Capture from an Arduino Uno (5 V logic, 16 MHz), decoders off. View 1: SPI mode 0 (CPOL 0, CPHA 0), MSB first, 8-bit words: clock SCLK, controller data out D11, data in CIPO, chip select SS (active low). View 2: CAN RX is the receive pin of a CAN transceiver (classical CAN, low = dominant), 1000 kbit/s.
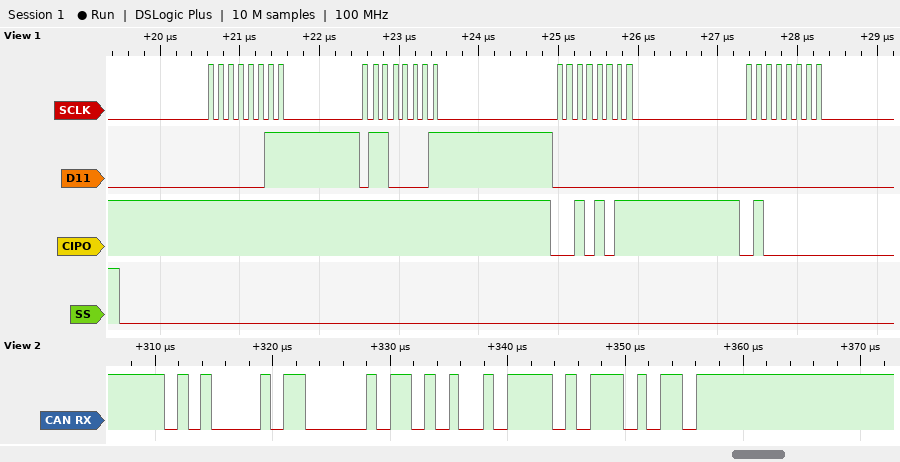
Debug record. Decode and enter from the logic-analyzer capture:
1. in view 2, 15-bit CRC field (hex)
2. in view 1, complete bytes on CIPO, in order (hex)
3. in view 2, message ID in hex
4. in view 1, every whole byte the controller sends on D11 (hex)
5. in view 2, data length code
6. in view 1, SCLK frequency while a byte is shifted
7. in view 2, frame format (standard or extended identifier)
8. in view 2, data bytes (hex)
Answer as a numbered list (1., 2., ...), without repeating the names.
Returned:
1. 0x3D75
2. 0xFF 0xFF 0x2B 0x40
3. 0x50B
4. 0x03 0x61 0x00 0x00
5. 1
6. 8 MHz
7. standard
8. A9
